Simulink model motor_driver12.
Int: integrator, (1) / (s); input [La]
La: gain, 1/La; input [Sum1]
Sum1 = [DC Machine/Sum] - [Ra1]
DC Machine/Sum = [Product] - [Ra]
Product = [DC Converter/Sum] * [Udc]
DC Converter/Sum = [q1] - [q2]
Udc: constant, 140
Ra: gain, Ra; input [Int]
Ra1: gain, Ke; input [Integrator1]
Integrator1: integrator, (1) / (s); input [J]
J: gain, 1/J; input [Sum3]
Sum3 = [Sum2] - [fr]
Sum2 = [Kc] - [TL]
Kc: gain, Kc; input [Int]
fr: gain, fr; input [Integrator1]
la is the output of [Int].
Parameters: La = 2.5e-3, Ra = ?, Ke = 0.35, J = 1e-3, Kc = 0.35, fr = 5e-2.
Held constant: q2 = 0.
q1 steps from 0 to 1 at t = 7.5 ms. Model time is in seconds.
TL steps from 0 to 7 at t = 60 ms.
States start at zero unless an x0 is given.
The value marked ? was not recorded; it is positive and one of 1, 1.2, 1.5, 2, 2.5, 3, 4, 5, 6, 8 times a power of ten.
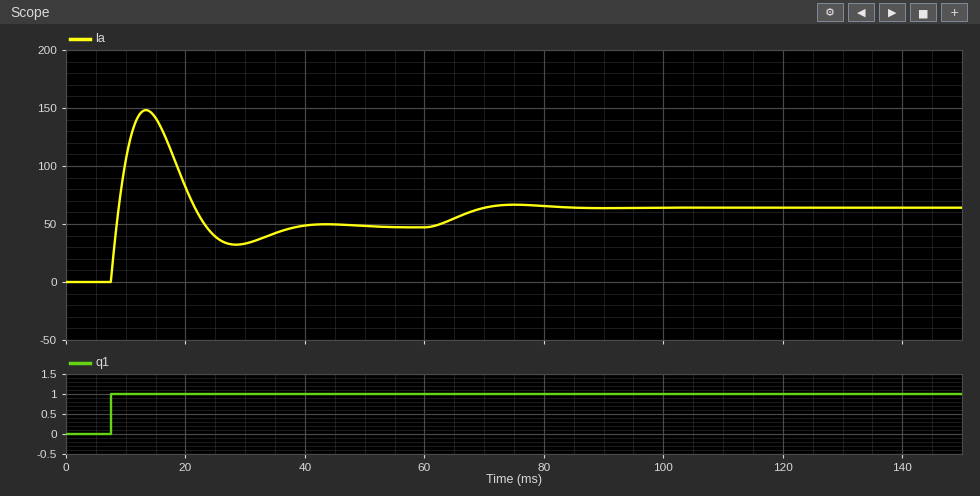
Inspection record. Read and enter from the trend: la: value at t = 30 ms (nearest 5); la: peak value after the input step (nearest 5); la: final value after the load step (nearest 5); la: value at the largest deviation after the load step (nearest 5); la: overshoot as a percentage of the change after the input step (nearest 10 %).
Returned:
35
150
65
65
210 %
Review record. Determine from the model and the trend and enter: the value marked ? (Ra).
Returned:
0.5
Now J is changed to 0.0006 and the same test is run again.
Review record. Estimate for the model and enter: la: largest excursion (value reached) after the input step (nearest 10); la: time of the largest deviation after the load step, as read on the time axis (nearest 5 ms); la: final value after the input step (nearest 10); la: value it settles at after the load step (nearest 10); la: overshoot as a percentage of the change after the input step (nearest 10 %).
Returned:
130
70 ms
50
60
170 %
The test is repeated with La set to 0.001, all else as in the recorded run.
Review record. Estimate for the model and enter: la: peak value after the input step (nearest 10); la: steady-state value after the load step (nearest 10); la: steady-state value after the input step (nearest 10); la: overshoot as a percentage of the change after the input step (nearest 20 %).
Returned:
180
60
50
280 %
